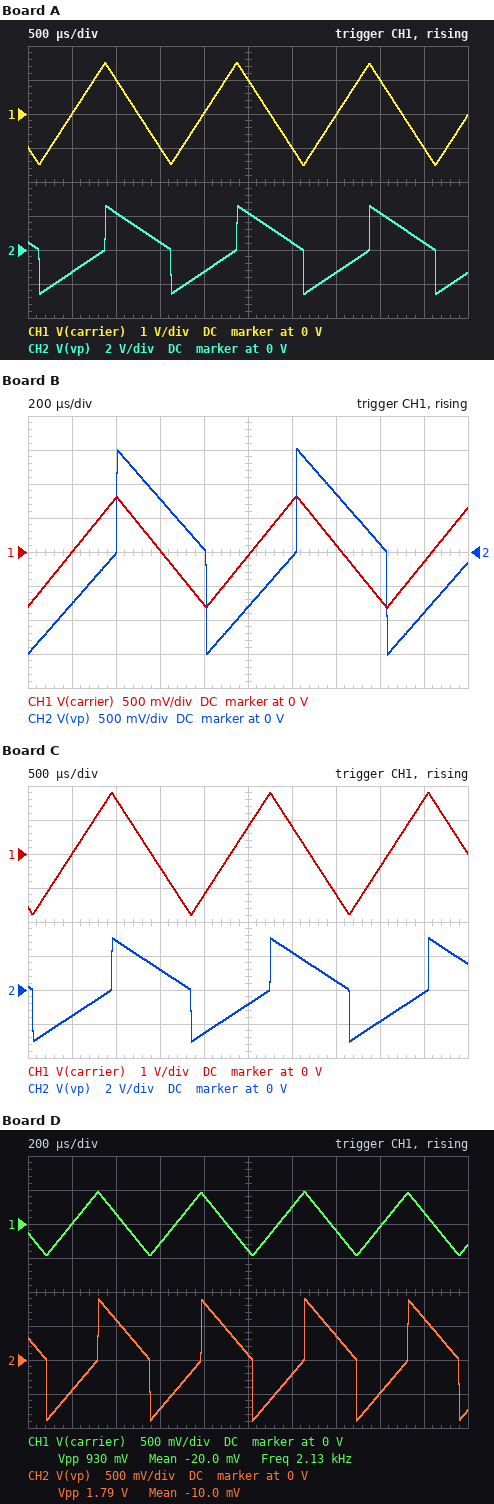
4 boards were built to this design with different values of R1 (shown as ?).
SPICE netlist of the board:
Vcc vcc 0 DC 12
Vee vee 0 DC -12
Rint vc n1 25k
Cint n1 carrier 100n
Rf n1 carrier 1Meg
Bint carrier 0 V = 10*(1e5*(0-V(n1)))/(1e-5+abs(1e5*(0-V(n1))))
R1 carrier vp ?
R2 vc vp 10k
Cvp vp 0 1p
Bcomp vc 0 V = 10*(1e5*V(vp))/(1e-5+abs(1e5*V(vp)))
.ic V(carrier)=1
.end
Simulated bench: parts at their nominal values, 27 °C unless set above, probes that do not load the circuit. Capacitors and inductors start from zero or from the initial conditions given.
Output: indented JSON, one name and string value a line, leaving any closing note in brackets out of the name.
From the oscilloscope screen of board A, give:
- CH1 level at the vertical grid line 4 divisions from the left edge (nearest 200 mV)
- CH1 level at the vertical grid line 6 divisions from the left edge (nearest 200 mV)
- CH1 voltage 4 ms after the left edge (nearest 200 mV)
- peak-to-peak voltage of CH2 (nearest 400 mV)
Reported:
{
  "CH1 level at the vertical grid line 4 divisions from the left edge": "0 V",
  "CH1 level at the vertical grid line 6 divisions from the left edge": "-1.0 V",
  "CH1 voltage 4 ms after the left edge": "1.0 V",
  "peak-to-peak voltage of CH2": "5.2 V"
}
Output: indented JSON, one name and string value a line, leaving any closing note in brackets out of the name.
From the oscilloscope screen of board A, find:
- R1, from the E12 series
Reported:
{
  "R1, from the E12 series": "1.5 kΩ"
}
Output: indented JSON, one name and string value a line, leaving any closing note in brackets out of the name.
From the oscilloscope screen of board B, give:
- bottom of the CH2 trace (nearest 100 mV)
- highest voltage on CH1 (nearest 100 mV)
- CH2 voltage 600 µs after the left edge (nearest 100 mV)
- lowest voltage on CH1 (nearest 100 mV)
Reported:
{
  "bottom of the CH2 trace": "-1.5 V",
  "highest voltage on CH1": "800 mV",
  "CH2 voltage 600 µs after the left edge": "800 mV",
  "lowest voltage on CH1": "-800 mV"
}
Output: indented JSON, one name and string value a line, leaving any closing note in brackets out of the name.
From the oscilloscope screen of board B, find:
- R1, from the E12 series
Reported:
{
  "R1, from the E12 series": "820 Ω"
}
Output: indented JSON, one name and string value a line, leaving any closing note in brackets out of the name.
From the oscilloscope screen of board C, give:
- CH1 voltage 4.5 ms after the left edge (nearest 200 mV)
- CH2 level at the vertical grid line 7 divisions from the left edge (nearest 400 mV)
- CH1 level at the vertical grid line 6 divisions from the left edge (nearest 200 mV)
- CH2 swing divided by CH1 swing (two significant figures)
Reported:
{
  "CH1 voltage 4.5 ms after the left edge": "1.6 V",
  "CH2 level at the vertical grid line 7 divisions from the left edge": "400 mV",
  "CH1 level at the vertical grid line 6 divisions from the left edge": "800 mV",
  "CH2 swing divided by CH1 swing": "1.7"
}
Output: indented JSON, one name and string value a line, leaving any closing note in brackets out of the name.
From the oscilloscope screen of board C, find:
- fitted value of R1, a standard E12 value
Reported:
{
  "fitted value of R1, a standard E12 value": "1.8 kΩ"
}
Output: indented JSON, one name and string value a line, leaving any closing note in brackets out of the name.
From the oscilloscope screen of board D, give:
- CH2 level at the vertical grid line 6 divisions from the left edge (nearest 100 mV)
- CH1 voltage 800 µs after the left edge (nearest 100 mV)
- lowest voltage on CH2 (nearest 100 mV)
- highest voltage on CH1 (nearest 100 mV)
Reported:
{
  "CH2 level at the vertical grid line 6 divisions from the left edge": "-200 mV",
  "CH1 voltage 800 µs after the left edge": "400 mV",
  "lowest voltage on CH2": "-900 mV",
  "highest voltage on CH1": "500 mV"
}
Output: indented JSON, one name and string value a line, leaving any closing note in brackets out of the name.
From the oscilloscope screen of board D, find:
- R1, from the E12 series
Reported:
{
  "R1, from the E12 series": "470 Ω"
}
